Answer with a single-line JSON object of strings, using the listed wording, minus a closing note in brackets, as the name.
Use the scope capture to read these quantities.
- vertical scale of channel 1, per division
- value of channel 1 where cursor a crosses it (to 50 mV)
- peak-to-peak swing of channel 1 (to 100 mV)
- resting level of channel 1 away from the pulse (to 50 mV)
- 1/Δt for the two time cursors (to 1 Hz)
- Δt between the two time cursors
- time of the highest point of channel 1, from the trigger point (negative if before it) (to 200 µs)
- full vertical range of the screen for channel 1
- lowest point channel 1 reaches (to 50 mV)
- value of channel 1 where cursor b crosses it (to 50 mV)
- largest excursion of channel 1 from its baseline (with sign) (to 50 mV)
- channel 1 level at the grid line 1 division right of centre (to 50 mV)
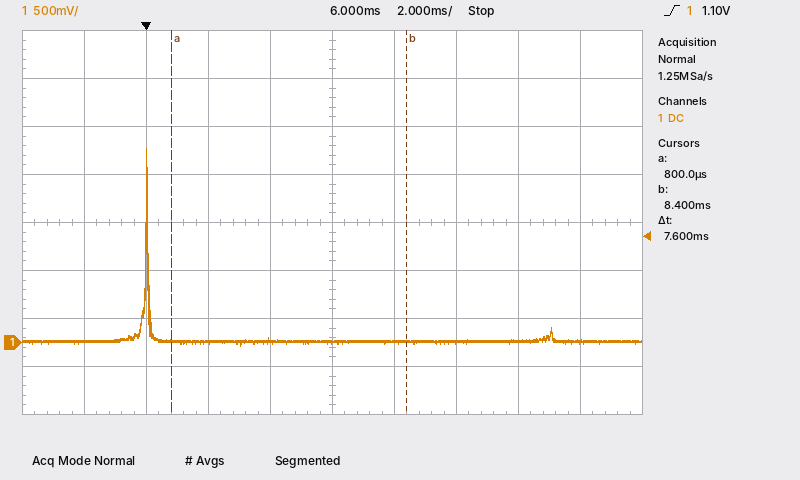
{"vertical scale of channel 1, per division": "500 mV", "value of channel 1 where cursor a crosses it": "0 mV", "peak-to-peak swing of channel 1": "2.10 V", "resting level of channel 1 away from the pulse": "0 mV", "1/Δt for the two time cursors": "132 Hz", "Δt between the two time cursors": "7.6 ms", "time of the highest point of channel 1, from the trigger point (negative if before it)": "0.0 ms", "full vertical range of the screen for channel 1": "4 V", "lowest point channel 1 reaches": "-50 mV", "value of channel 1 where cursor b crosses it": "0 mV", "largest excursion of channel 1 from its baseline (with sign)": "+2.00 V", "channel 1 level at the grid line 1 division right of centre": "0 mV"}
